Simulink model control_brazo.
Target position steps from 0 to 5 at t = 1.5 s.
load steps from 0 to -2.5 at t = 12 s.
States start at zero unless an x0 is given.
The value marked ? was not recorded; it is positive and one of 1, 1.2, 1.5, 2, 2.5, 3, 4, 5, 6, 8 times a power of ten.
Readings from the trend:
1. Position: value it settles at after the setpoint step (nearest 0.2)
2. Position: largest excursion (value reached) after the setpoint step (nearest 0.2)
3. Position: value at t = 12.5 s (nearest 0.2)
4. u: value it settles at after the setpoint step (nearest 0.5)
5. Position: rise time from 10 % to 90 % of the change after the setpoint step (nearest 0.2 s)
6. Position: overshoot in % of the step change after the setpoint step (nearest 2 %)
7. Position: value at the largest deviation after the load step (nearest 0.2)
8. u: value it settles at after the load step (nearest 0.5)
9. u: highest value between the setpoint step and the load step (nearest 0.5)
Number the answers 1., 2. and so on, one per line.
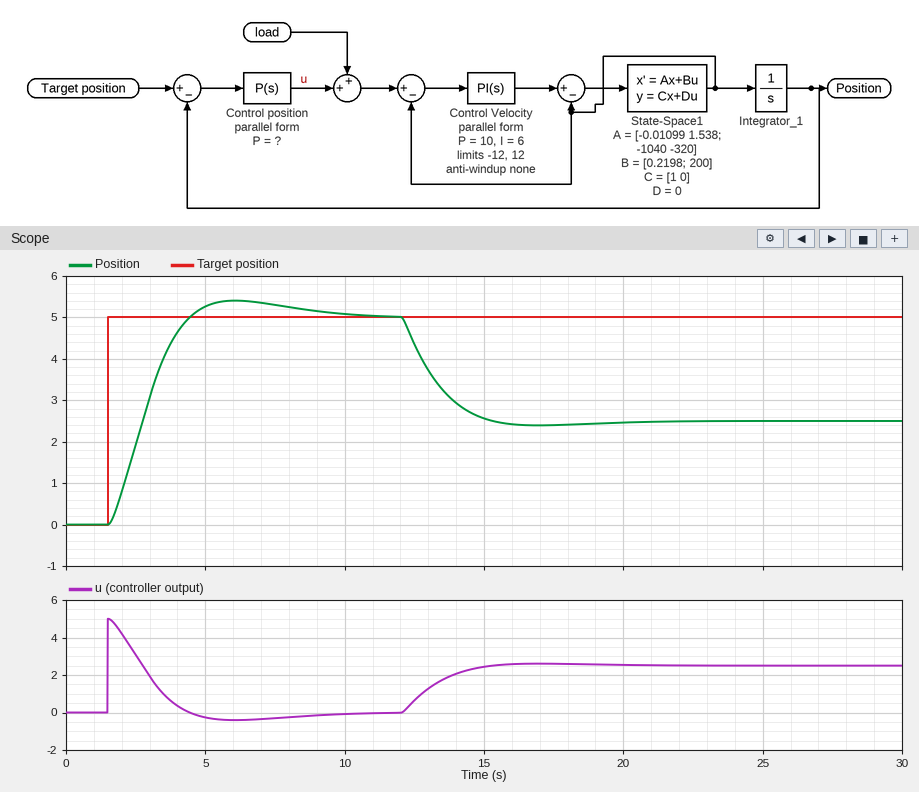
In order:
1. 5.0
2. 5.4
3. 4.4
4. 0.0
5. 2.0 s
6. 8 %
7. 2.4
8. 2.5
9. 5.0
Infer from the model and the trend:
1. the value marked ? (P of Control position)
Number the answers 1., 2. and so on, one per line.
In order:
1. 1
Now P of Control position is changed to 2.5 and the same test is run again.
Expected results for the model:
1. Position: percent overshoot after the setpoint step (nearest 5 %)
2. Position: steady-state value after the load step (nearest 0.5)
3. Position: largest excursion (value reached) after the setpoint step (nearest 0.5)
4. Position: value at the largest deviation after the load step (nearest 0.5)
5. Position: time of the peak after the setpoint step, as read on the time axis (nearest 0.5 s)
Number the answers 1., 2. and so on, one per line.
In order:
1. 30 %
2. 4.0
3. 6.5
4. 4.0
5. 5.0 s
